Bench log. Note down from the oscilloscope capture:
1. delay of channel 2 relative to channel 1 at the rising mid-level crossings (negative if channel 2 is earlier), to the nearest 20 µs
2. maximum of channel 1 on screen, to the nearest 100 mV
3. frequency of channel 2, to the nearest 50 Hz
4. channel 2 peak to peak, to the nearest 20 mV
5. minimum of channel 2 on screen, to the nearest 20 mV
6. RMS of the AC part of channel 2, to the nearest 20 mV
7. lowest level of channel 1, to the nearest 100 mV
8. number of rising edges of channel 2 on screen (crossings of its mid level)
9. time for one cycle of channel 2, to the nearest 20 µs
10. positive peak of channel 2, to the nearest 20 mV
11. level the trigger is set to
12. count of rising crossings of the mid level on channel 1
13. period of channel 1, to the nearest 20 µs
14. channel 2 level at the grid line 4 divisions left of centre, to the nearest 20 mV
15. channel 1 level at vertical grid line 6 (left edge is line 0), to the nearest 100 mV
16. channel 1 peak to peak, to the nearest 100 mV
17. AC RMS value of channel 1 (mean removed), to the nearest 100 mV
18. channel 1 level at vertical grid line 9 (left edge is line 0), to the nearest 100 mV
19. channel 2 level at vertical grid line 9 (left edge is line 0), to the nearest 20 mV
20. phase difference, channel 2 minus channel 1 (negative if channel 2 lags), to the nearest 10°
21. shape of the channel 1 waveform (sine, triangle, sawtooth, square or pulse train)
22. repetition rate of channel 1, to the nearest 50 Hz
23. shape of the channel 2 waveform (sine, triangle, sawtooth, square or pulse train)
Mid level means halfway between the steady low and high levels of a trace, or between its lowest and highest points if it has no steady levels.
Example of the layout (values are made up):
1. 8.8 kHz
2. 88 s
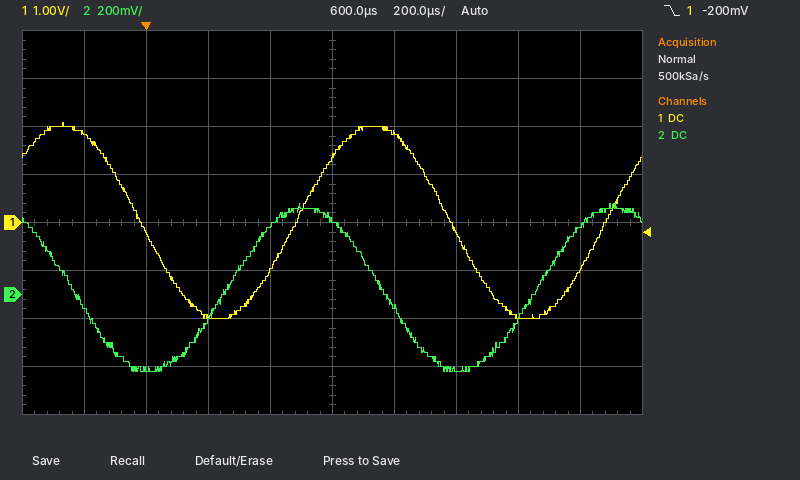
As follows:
1. -220 µs
2. 2.1 V
3. 1.00 kHz
4. 700 mV
5. -320 mV
6. 240 mV
7. -2.0 V
8. 2
9. 1.00 ms
10. 380 mV
11. -200 mV
12. 2
13. 1.00 ms
14. -60 mV
15. 1.9 V
16. 4.1 V
17. 1.4 V
18. -1.0 V
19. 280 mV
20. +80°
21. sine
22. 1.00 kHz
23. sine
